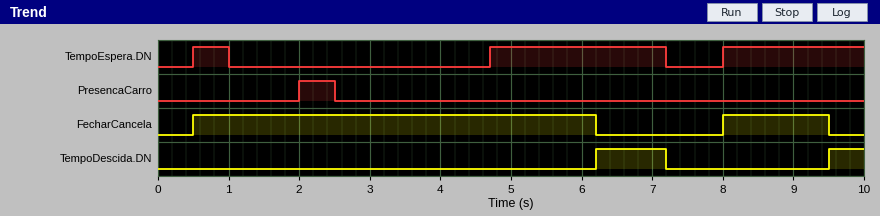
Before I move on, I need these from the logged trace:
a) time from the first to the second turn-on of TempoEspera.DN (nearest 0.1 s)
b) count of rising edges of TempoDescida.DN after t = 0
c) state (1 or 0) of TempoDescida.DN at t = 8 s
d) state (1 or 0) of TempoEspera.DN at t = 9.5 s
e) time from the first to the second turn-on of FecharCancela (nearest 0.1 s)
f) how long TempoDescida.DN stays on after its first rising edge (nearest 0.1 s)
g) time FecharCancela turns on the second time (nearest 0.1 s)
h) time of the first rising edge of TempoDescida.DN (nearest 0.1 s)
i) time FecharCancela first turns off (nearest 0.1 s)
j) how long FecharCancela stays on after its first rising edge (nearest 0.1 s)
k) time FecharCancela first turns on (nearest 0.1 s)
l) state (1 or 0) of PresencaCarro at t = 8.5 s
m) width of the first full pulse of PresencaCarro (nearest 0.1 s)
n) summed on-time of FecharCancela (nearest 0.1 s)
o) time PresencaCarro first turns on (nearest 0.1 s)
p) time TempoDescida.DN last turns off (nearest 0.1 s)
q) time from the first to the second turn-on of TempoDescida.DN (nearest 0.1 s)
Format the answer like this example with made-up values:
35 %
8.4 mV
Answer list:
4.2 s
2
0
1
7.5 s
1.0 s
8.0 s
6.2 s
6.2 s
5.7 s
0.5 s
0
0.5 s
7.2 s
2.0 s
7.2 s
3.3 s
